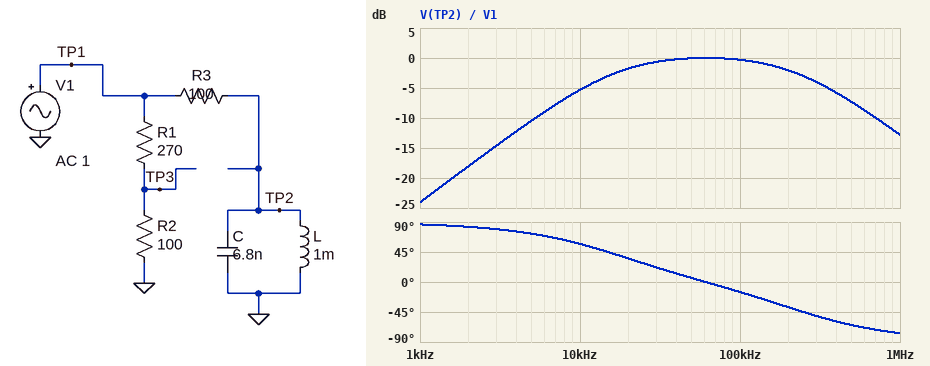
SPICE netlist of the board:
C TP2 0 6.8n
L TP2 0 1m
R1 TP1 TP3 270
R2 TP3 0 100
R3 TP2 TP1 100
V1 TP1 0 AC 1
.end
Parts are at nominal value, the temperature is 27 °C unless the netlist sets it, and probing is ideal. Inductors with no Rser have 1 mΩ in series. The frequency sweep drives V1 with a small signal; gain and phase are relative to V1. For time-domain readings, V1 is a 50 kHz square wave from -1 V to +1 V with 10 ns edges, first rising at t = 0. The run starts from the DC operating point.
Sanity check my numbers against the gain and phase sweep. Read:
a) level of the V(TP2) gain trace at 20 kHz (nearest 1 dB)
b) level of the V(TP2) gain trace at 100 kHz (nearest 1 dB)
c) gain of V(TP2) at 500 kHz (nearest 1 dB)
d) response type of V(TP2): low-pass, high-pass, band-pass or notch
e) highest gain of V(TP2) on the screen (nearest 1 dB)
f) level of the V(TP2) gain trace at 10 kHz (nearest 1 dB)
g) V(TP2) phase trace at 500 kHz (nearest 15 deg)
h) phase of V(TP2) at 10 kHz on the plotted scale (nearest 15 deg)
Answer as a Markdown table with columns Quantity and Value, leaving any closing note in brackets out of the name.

| Quantity | Value |
|---|---|
| level of the V(TP2) gain trace at 20 kHz | -2 dB |
| level of the V(TP2) gain trace at 100 kHz | 0 dB |
| gain of V(TP2) at 500 kHz | -7 dB |
| response type of V(TP2): low-pass, high-pass, band-pass or notch | band-pass |
| highest gain of V(TP2) on the screen | 0 dB |
| level of the V(TP2) gain trace at 10 kHz | -5 dB |
| V(TP2) phase trace at 500 kHz | -60 deg |
| phase of V(TP2) at 10 kHz on the plotted scale | 60 deg |
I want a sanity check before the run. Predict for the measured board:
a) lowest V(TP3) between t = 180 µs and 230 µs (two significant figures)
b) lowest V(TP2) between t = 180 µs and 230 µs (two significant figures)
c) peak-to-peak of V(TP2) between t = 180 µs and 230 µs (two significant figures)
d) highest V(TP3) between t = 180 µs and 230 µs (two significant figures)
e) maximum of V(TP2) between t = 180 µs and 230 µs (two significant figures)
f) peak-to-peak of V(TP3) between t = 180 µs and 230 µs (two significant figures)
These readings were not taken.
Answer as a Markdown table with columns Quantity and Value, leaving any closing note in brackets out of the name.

| Quantity | Value |
|---|---|
| lowest V(TP3) between t = 180 µs and 230 µs | -270 mV |
| lowest V(TP2) between t = 180 µs and 230 µs | -1.3 V |
| peak-to-peak of V(TP2) between t = 180 µs and 230 µs | 2.5 V |
| highest V(TP3) between t = 180 µs and 230 µs | 270 mV |
| maximum of V(TP2) between t = 180 µs and 230 µs | 1.3 V |
| peak-to-peak of V(TP3) between t = 180 µs and 230 µs | 540 mV |
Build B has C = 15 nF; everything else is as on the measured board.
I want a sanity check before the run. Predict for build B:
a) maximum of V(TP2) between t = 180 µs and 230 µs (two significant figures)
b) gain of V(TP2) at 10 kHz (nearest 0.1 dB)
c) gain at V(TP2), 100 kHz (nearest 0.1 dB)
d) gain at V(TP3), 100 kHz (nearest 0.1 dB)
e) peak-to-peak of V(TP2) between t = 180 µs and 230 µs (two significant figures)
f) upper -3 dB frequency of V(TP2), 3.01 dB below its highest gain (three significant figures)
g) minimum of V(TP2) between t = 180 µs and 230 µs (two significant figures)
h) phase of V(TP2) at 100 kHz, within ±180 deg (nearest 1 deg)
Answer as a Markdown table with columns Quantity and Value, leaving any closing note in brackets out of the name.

| Quantity | Value |
|---|---|
| maximum of V(TP2) between t = 180 µs and 230 µs | 1.1 V |
| gain of V(TP2) at 10 kHz | -5.1 dB |
| gain at V(TP2), 100 kHz | -2.1 dB |
| gain at V(TP3), 100 kHz | -11.4 dB |
| peak-to-peak of V(TP2) between t = 180 µs and 230 µs | 2.3 V |
| upper -3 dB frequency of V(TP2), 3.01 dB below its highest gain | 120 kHz |
| minimum of V(TP2) between t = 180 µs and 230 µs | -1.1 V |
| phase of V(TP2) at 100 kHz, within ±180 deg | -38 deg |
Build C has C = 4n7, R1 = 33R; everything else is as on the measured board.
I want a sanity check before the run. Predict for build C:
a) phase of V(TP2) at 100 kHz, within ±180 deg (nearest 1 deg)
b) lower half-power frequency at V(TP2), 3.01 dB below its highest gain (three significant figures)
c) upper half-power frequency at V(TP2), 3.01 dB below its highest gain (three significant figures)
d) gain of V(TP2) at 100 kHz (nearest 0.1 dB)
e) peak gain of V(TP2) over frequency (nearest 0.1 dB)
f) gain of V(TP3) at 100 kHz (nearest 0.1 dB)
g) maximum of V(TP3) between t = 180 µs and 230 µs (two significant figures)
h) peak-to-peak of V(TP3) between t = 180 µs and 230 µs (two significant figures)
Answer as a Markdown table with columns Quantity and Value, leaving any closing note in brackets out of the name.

| Quantity | Value |
|---|---|
| phase of V(TP2) at 100 kHz, within ±180 deg | -8 deg |
| lower half-power frequency at V(TP2), 3.01 dB below its highest gain | 15.2 kHz |
| upper half-power frequency at V(TP2), 3.01 dB below its highest gain | 354 kHz |
| gain of V(TP2) at 100 kHz | -0.1 dB |
| peak gain of V(TP2) over frequency | 0 dB |
| gain of V(TP3) at 100 kHz | -2.5 dB |
| maximum of V(TP3) between t = 180 µs and 230 µs | 750 mV |
| peak-to-peak of V(TP3) between t = 180 µs and 230 µs | 1.5 V |
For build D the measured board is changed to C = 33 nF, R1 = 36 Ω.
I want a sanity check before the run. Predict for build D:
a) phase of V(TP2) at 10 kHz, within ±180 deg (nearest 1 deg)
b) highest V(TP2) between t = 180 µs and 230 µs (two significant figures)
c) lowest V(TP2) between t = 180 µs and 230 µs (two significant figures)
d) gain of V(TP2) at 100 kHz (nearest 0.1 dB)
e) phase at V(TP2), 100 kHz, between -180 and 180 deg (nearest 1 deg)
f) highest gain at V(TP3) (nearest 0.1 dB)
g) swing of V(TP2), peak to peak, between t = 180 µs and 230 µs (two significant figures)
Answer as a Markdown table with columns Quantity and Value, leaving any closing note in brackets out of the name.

| Quantity | Value |
|---|---|
| phase of V(TP2) at 10 kHz, within ±180 deg | 54 deg |
| highest V(TP2) between t = 180 µs and 230 µs | 940 mV |
| lowest V(TP2) between t = 180 µs and 230 µs | -940 mV |
| gain of V(TP2) at 100 kHz | -6.7 dB |
| phase at V(TP2), 100 kHz, between -180 and 180 deg | -62 deg |
| highest gain at V(TP3) | -2.7 dB |
| swing of V(TP2), peak to peak, between t = 180 µs and 230 µs | 1.9 V |
